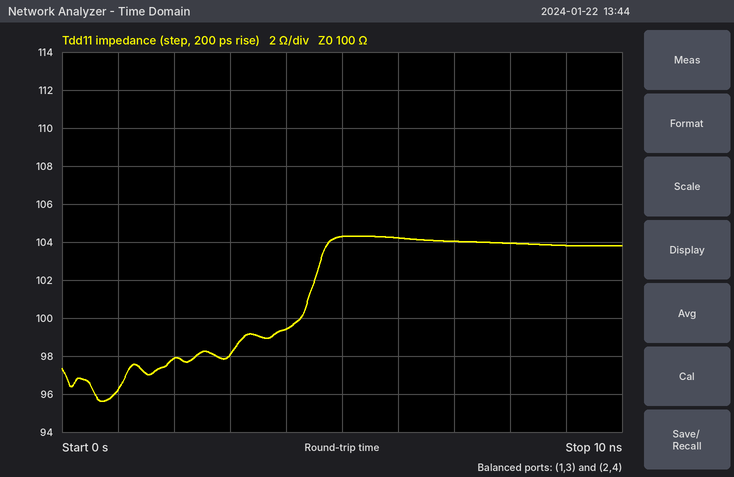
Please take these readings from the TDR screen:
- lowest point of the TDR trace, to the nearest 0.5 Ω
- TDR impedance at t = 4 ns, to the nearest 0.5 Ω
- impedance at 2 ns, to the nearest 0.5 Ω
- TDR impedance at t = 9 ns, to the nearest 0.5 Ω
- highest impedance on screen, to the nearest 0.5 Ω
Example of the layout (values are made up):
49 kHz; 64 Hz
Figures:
95.5 Ω; 99.5 Ω; 98.0 Ω; 104.0 Ω; 104.5 Ω
